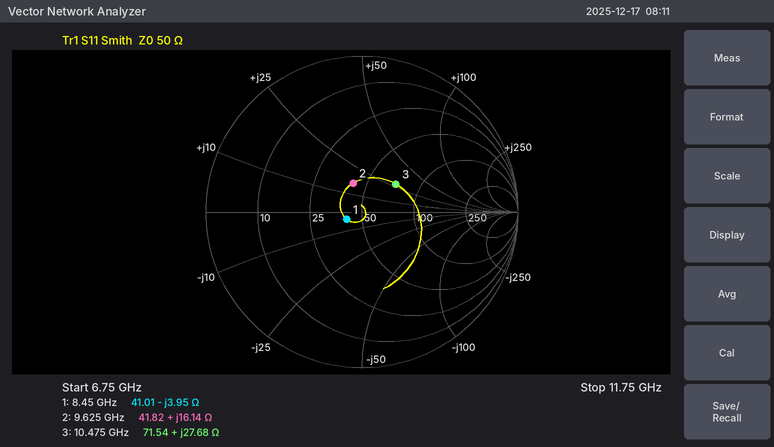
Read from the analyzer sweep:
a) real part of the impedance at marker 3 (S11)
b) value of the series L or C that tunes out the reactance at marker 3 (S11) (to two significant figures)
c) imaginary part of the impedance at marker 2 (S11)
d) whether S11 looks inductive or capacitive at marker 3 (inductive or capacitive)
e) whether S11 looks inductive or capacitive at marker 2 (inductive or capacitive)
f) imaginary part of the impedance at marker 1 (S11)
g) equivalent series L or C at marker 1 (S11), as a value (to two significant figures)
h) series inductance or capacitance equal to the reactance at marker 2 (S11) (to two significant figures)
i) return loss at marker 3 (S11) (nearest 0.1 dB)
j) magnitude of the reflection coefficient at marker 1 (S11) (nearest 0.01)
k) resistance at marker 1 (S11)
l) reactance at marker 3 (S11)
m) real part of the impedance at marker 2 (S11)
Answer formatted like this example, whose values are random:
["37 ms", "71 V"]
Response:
["71.54 Ω", "550 fF", "+16.14 Ω", "inductive", "inductive", "-3.95 Ω", "4.8 pF", "270 pH", "11.0 dB", "0.11", "41.01 Ω", "+27.68 Ω", "41.82 Ω"]
